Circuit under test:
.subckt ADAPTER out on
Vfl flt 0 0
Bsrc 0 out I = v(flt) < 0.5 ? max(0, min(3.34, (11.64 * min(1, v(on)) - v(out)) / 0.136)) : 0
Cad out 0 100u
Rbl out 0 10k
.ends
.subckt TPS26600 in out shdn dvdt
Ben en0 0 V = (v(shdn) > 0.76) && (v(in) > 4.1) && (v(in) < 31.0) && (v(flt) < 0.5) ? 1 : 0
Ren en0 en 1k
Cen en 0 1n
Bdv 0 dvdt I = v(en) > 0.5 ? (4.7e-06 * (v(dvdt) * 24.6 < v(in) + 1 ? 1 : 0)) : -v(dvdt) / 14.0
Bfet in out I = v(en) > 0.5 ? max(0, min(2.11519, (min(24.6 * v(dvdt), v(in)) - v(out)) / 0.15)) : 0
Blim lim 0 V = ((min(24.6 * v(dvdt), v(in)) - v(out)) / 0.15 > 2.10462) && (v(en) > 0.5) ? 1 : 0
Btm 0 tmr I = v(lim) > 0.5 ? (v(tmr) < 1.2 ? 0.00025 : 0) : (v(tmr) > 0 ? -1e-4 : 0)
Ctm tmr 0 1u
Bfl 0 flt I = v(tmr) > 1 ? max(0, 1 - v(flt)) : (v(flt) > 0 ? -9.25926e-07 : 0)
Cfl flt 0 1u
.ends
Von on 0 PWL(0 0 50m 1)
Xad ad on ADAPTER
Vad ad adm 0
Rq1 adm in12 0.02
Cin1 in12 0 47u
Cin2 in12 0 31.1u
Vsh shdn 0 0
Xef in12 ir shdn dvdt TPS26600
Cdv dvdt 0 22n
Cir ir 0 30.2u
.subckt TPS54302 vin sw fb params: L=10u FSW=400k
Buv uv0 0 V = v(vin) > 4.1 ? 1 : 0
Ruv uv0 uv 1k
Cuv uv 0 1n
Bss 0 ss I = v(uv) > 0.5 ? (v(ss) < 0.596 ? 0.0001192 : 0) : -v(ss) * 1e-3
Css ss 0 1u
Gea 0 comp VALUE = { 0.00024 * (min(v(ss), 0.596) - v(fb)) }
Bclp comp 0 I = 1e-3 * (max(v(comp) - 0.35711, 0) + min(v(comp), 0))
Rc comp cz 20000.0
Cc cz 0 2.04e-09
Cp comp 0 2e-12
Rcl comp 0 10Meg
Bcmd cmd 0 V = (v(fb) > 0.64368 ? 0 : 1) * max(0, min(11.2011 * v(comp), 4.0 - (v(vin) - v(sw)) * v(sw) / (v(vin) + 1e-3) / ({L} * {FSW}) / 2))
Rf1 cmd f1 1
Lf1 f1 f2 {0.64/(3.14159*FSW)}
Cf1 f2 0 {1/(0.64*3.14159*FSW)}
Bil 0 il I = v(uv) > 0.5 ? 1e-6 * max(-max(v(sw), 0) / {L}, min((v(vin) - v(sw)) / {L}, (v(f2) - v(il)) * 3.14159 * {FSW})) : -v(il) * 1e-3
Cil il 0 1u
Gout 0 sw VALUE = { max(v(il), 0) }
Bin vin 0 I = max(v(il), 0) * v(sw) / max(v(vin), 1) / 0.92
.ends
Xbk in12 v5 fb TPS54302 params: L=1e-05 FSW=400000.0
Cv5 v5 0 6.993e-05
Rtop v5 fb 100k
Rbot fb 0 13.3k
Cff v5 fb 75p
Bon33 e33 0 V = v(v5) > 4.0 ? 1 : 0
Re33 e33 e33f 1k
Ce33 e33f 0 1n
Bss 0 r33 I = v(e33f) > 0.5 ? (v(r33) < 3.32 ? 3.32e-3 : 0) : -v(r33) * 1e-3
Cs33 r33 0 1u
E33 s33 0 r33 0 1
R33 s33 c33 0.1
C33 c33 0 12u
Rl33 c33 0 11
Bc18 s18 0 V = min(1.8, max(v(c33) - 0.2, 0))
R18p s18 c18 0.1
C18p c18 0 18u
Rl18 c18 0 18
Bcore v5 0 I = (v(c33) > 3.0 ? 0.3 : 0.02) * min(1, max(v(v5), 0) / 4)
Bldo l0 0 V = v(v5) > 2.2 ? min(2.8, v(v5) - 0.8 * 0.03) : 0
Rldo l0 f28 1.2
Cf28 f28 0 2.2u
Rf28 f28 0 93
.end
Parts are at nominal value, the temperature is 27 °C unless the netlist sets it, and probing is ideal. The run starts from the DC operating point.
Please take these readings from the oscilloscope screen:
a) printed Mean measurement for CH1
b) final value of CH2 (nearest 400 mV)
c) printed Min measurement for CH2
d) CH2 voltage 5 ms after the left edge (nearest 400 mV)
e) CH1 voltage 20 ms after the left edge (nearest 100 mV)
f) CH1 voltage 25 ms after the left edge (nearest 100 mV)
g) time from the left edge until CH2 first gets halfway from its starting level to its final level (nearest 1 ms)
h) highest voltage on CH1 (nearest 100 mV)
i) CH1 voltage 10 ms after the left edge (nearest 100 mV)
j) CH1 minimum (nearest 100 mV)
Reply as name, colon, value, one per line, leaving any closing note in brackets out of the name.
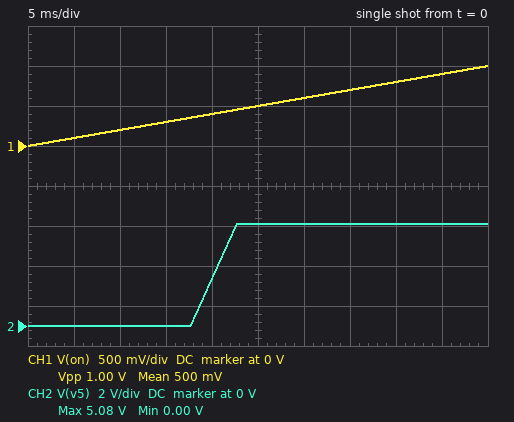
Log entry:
printed Mean measurement for CH1: 500 mV
final value of CH2: 5.2 V
printed Min measurement for CH2: 0.00 V
CH2 voltage 5 ms after the left edge: 0 V
CH1 voltage 20 ms after the left edge: 400 mV
CH1 voltage 25 ms after the left edge: 500 mV
time from the left edge until CH2 first gets halfway from its starting level to its final level: 20 ms
highest voltage on CH1: 1.0 V
CH1 voltage 10 ms after the left edge: 200 mV
CH1 minimum: 0 V
